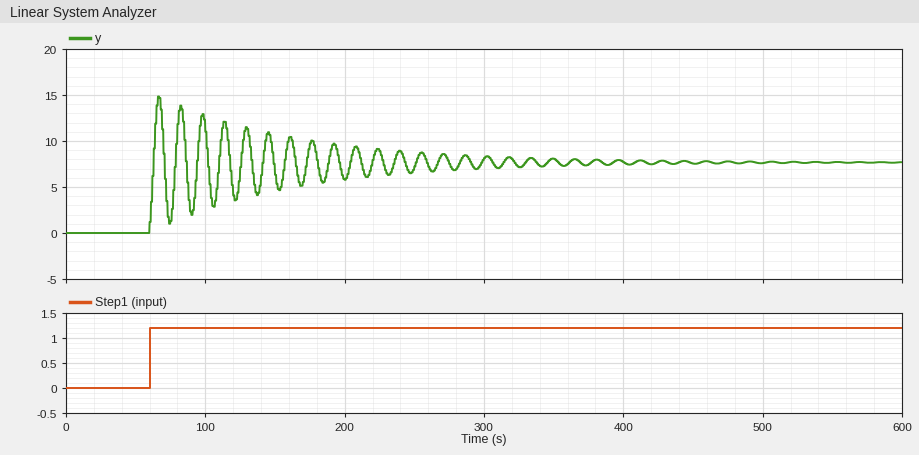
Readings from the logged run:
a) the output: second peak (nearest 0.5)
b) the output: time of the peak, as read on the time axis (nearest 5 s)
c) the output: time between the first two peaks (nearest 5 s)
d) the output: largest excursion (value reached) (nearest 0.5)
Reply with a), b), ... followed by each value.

a) 14.0
b) 65 s
c) 15 s
d) 15.0
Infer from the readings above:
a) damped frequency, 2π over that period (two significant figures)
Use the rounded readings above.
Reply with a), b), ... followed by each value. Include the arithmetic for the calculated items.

a) 2π / 15 = 0.42 rad/s
